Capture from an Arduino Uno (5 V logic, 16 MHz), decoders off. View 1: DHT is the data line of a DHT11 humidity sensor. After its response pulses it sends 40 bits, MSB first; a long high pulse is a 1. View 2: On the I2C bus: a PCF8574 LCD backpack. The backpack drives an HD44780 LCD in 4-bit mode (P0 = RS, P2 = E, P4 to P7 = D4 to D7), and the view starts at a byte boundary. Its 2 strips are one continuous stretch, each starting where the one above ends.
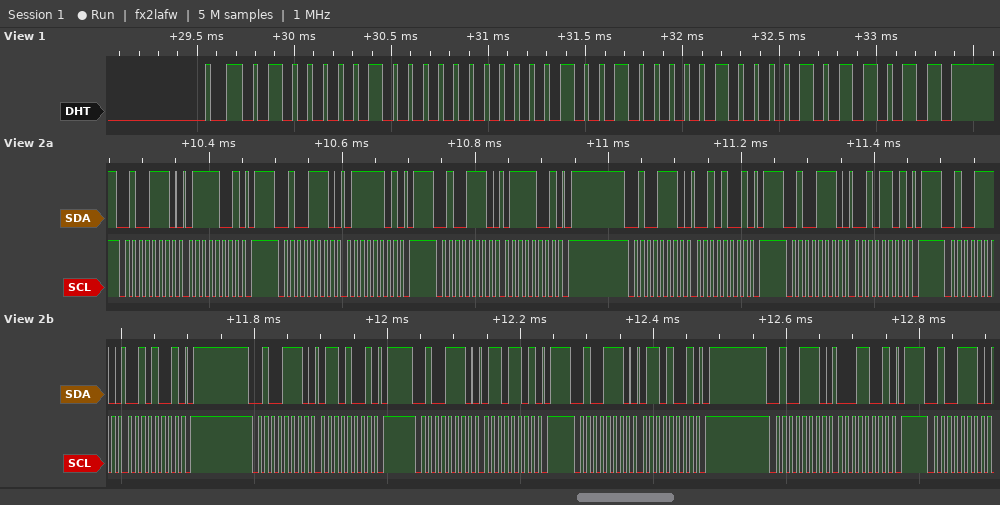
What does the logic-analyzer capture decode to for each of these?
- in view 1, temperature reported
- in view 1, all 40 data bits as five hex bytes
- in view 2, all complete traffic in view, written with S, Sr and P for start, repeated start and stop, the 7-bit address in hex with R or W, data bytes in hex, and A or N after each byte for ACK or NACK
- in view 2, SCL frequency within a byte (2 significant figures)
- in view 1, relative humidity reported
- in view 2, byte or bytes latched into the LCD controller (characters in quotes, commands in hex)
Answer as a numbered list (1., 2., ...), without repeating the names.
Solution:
1. 18.8 °C
2. 41 00 12 08 5B
3. S 27W A 79 A P S 27W A 7D A P S 27W A 79 A P S 27W A 29 A P S 27W A 2D A P S 27W A 29 A P S 27W A 69 A P S 27W A 6D A P S 27W A 69 A P S 27W A 19 A P S 27W A
4. 100 kHz
5. 65 %
6. 'r'
